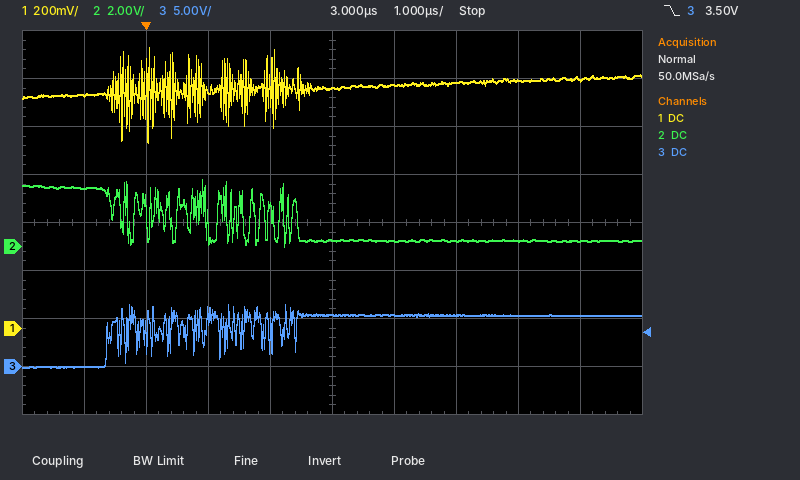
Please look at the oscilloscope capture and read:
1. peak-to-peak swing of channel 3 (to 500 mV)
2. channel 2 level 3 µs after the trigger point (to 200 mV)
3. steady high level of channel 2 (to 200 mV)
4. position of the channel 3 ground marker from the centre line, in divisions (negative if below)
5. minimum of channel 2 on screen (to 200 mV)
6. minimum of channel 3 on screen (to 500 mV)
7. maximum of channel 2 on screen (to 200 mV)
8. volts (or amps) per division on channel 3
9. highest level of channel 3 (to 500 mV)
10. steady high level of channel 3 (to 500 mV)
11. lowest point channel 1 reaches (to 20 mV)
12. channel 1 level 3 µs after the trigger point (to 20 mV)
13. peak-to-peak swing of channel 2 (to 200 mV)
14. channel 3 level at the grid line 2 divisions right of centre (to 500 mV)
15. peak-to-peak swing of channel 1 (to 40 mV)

6.5 V
200 mV
2.4 V
-3.0 div
0.0 V
0.0 V
2.8 V
5 V
6.5 V
5.5 V
780 mV
1.00 V
2.8 V
5.5 V
400 mV
